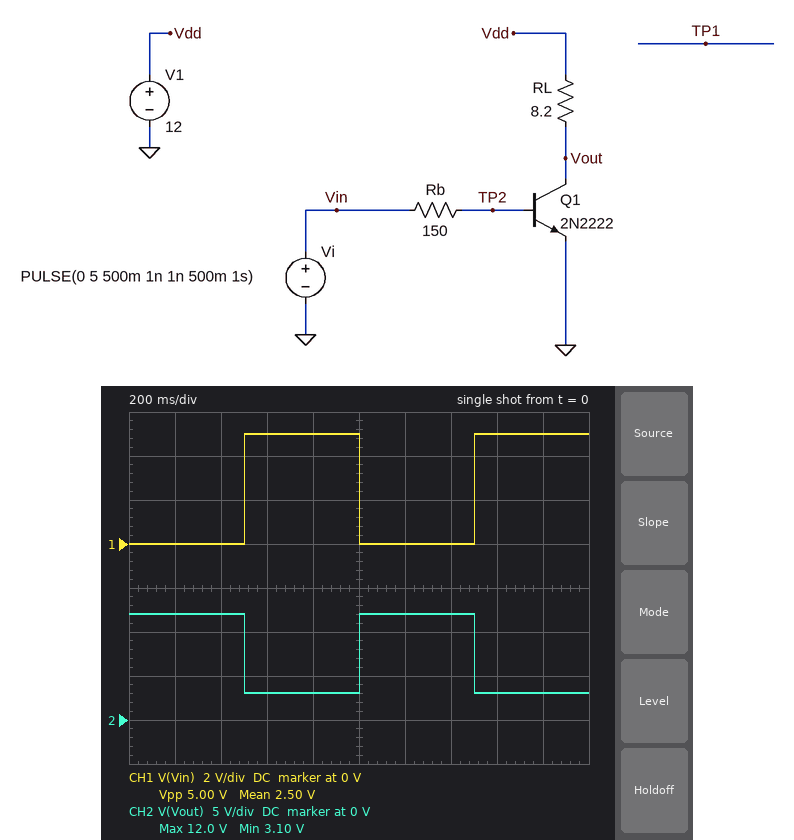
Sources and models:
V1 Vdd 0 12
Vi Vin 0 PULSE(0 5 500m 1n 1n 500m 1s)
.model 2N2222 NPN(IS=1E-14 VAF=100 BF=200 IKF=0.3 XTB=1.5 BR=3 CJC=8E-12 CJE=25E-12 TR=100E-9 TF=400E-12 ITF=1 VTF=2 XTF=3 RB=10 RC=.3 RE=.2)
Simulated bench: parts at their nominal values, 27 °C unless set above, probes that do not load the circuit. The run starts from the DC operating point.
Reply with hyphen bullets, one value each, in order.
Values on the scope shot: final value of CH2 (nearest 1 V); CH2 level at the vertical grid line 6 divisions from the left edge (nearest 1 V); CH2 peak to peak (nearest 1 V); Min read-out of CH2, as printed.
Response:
- 3 V
- 12 V
- 9 V
- 3.10 V
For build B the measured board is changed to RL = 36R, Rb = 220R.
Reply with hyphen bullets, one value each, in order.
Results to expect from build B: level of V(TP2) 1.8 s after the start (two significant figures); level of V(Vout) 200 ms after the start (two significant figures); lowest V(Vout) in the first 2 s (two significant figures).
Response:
- 1.1 V
- 12 V
- 240 mV
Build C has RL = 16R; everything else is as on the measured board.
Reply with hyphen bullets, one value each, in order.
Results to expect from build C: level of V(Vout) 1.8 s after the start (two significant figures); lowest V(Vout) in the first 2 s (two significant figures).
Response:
- 480 mV
- 470 mV
